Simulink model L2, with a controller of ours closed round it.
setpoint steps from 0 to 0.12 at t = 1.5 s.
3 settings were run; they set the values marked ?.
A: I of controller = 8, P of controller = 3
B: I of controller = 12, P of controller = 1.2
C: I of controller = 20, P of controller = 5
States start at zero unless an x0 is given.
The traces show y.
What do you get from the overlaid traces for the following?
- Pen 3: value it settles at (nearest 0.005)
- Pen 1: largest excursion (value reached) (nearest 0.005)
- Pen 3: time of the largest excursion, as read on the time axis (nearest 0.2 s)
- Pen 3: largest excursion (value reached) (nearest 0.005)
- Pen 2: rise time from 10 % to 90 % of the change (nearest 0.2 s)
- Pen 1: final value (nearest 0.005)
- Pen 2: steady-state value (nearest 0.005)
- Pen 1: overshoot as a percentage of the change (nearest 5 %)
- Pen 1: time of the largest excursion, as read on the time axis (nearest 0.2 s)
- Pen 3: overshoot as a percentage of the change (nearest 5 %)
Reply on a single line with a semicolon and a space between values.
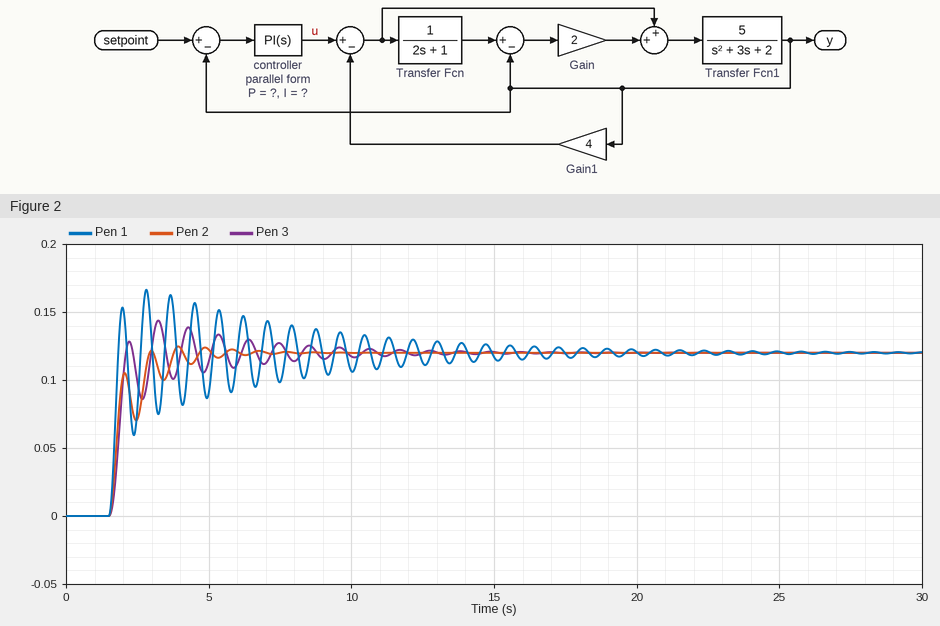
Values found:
0.120; 0.165; 3.2 s; 0.145; 1.2 s; 0.120; 0.120; 40 %; 2.8 s; 20 %
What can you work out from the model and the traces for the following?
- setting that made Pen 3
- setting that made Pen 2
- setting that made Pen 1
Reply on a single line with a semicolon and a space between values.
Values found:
B; A; C
